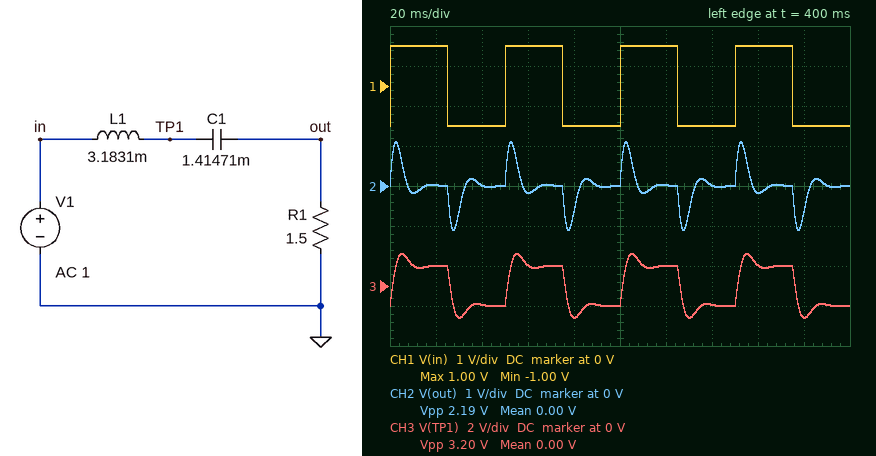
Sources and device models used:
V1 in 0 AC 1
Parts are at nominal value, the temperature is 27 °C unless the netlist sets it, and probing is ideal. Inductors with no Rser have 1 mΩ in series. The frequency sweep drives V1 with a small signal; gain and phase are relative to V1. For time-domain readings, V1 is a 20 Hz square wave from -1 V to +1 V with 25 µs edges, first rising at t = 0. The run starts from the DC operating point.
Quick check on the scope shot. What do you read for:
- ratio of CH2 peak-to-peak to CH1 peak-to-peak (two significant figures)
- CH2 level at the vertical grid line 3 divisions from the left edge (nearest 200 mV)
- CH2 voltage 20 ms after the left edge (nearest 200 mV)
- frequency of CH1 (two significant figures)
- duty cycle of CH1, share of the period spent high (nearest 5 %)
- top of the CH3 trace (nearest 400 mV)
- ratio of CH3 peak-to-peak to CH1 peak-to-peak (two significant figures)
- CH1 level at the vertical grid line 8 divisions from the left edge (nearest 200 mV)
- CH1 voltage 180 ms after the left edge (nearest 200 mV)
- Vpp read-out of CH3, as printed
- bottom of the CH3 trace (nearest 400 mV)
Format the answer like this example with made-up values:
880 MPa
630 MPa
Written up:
1.1
-200 mV
0 V
20 Hz
50 %
1.6 V
1.6
1.0 V
-1.0 V
3.20 V
-1.6 V
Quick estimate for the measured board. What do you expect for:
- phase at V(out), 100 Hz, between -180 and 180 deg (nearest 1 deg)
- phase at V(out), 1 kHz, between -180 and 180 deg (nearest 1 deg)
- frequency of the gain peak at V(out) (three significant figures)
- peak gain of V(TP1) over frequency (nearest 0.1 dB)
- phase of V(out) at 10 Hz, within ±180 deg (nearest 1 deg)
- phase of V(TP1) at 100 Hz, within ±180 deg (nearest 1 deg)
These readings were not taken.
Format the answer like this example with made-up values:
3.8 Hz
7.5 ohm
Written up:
-30 deg
-86 deg
75.0 Hz
3.3 dB
82 deg
-67 deg
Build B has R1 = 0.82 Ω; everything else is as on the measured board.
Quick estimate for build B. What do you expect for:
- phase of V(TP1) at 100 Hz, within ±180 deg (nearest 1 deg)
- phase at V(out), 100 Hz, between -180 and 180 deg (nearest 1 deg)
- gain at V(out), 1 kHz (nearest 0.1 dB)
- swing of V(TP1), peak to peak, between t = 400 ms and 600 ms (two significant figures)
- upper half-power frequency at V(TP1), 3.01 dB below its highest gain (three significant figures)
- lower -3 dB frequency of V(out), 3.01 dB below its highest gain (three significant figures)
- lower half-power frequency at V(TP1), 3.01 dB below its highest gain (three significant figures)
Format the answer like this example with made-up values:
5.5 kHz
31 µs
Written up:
-101 deg
-47 deg
-27.7 dB
3.9 V
90.1 Hz
57.2 Hz
46.7 Hz
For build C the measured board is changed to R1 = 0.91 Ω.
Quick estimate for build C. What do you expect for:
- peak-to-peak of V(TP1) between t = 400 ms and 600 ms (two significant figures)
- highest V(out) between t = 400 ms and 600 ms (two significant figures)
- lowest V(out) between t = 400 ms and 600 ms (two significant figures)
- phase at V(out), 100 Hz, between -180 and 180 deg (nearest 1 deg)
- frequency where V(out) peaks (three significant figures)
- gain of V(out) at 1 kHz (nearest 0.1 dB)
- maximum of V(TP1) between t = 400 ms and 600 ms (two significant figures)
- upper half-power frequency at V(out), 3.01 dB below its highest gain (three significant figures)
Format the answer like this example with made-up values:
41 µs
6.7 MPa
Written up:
3.8 V
810 mV
-810 mV
-44 deg
75.0 Hz
-26.8 dB
1.9 V
101 Hz
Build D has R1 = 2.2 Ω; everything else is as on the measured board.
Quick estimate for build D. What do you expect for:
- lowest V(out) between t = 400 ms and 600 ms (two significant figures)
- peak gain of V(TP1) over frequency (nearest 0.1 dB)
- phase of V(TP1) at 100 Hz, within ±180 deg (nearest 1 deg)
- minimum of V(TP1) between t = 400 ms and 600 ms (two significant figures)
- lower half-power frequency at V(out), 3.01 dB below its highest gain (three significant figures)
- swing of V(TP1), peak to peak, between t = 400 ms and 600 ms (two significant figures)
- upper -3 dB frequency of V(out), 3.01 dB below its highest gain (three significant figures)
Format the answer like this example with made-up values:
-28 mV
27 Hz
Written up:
-1.3 V
2.0 dB
-49 deg
-1.4 V
38.0 Hz
2.8 V
148 Hz
